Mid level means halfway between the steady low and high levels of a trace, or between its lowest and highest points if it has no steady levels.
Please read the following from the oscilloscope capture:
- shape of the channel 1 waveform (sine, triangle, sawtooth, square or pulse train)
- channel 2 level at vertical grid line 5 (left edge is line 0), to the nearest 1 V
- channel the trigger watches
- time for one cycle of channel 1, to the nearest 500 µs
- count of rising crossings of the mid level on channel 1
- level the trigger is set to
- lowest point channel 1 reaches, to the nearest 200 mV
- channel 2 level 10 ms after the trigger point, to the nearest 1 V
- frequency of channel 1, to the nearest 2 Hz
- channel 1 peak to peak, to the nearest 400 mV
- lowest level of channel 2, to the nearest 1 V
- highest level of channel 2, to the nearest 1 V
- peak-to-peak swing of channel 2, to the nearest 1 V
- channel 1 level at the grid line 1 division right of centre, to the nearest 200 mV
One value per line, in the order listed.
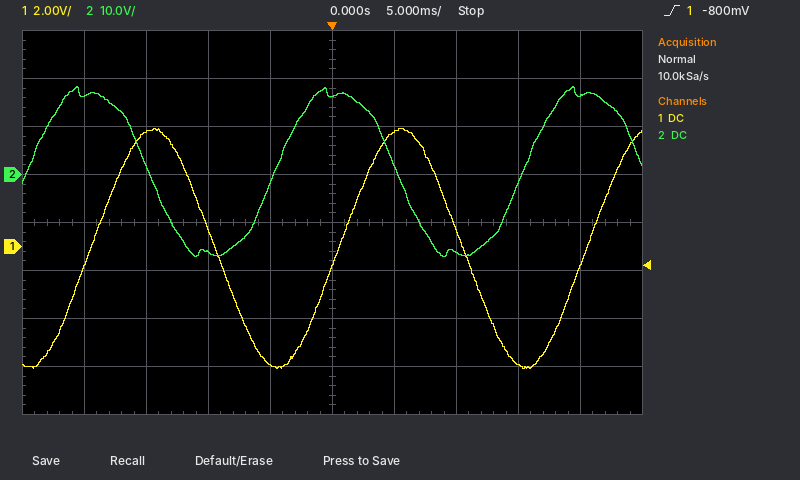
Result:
sine
16 V
channel 1
20.0 ms
3
-800 mV
-5.0 V
-16 V
50 Hz
10.0 V
-17 V
18 V
35 V
4.8 V
